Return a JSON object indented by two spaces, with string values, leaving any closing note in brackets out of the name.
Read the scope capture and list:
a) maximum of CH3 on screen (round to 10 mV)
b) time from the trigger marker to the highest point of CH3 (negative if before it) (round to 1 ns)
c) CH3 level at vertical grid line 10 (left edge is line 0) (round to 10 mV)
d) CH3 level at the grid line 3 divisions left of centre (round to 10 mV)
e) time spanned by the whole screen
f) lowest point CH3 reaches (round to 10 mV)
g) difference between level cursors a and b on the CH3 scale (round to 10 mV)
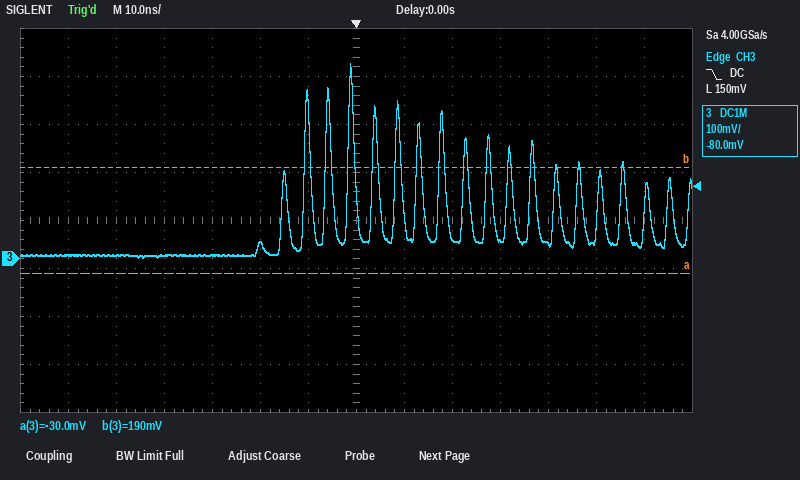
{
  "maximum of CH3 on screen": "410 mV",
  "time from the trigger marker to the highest point of CH3 (negative if before it)": "-1 ns",
  "CH3 level at vertical grid line 10 (left edge is line 0)": "40 mV",
  "CH3 level at the grid line 3 divisions left of centre": "10 mV",
  "time spanned by the whole screen": "140 ns",
  "lowest point CH3 reaches": "0 mV",
  "difference between level cursors a and b on the CH3 scale": "220 mV"
}
